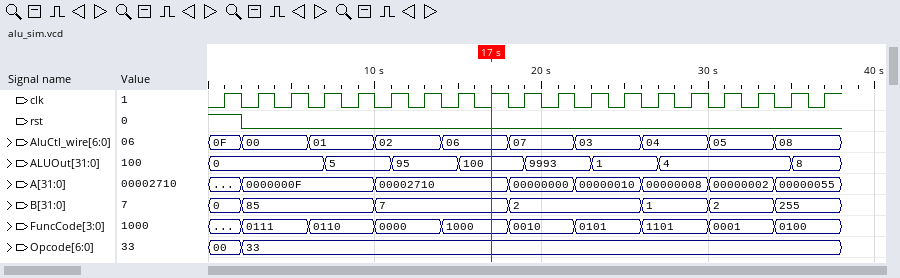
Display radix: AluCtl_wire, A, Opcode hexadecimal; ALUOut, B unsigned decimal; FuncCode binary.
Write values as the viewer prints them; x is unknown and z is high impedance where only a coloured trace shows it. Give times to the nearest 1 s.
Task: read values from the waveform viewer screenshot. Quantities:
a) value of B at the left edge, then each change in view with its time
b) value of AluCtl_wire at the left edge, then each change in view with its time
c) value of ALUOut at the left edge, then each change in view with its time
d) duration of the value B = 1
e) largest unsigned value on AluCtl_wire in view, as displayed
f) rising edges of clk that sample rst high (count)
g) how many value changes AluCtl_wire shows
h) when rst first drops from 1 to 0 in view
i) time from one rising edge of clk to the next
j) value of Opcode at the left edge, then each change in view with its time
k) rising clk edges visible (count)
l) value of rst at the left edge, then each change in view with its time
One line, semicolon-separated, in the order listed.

0, 85 at 2 s, 7 at 10 s, 2 at 18 s, 1 at 26 s, 2 at 30 s, 255 at 34 s; 0F, 00 at 2 s, 01 at 6 s, 02 at 10 s, 06 at 14 s, 07 at 18 s, 03 at 22 s, 04 at 26 s, 05 at 30 s, 08 at 34 s; 0, 5 at 7 s, 95 at 11 s, 100 at 15 s, 9993 at 19 s, 1 at 23 s, 4 at 27 s, 8 at 35 s; 4 s; 0F; 1; 9; 2 s; 2 s; 00, 33 at 2 s; 19; 1, 0 at 2 s
